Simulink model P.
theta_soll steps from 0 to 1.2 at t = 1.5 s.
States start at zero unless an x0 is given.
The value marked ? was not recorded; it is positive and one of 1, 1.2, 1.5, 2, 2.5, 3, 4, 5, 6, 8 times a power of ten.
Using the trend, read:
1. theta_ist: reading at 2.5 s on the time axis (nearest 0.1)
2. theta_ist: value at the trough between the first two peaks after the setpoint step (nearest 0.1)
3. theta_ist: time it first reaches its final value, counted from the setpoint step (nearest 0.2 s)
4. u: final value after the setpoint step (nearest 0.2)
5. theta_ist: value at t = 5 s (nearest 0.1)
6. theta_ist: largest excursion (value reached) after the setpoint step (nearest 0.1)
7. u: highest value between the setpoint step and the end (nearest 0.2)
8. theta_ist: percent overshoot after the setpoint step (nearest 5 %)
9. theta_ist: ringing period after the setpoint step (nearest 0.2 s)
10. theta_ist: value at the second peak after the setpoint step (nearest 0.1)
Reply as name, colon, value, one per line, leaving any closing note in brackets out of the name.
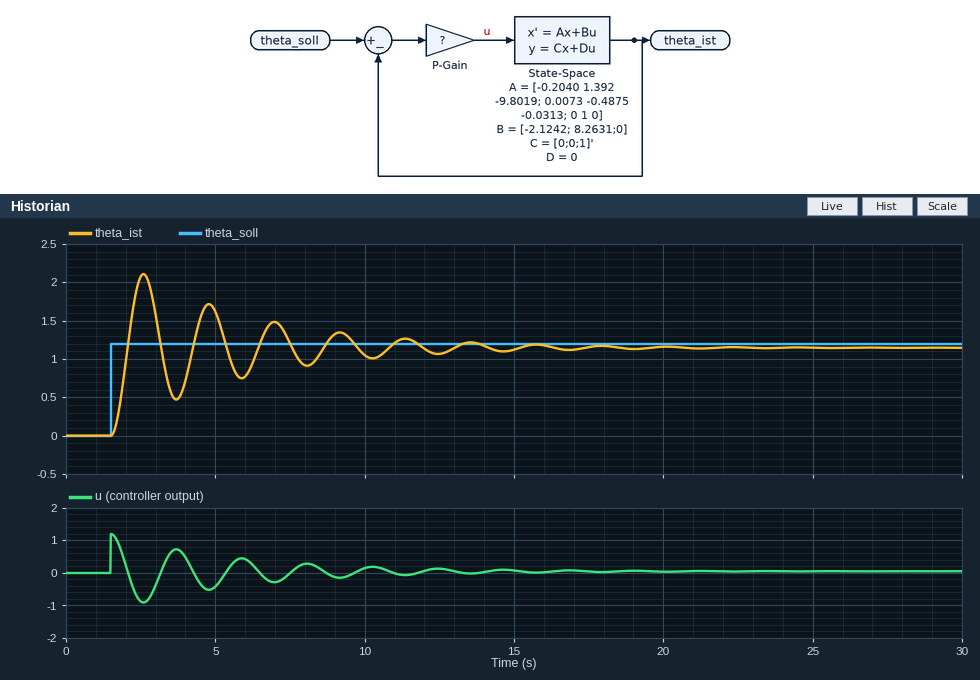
theta_ist: reading at 2.5 s on the time axis: 2.1
theta_ist: value at the trough between the first two peaks after the setpoint step: 0.5
theta_ist: time it first reaches its final value, counted from the setpoint step: 0.6 s
u: final value after the setpoint step: 0.0
theta_ist: value at t = 5 s: 1.6
theta_ist: largest excursion (value reached) after the setpoint step: 2.1
u: highest value between the setpoint step and the end: 1.2
theta_ist: percent overshoot after the setpoint step: 85 %
theta_ist: ringing period after the setpoint step: 2.2 s
theta_ist: value at the second peak after the setpoint step: 1.7
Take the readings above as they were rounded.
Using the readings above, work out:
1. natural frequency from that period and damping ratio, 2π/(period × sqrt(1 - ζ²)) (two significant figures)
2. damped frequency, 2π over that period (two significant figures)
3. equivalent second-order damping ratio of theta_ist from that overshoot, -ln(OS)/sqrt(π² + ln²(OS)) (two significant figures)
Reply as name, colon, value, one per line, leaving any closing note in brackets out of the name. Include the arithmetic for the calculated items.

natural frequency from that period and damping ratio, 2π/(period × sqrt(1 - ζ²)): 2π / (2.2 × sqrt(1 - 0.052²)) = 2.9 rad/s
damped frequency, 2π over that period: 2π / 2.2 = 2.9 rad/s
equivalent second-order damping ratio of theta_ist from that overshoot, -ln(OS)/sqrt(π² + ln²(OS)): ln(0.85) = -0.163; 0.163 / sqrt(9.870 + 0.026) = 0.052
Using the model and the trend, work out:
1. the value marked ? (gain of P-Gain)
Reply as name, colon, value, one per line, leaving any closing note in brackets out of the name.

the value marked ?: 1
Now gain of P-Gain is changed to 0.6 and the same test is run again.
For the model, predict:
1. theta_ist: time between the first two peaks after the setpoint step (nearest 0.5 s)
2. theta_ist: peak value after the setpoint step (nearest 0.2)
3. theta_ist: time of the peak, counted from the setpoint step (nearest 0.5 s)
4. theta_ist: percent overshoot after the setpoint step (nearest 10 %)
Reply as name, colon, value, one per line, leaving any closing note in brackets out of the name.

theta_ist: time between the first two peaks after the setpoint step: 3.0 s
theta_ist: peak value after the setpoint step: 2.0
theta_ist: time of the peak, counted from the setpoint step: 1.5 s
theta_ist: percent overshoot after the setpoint step: 80 %
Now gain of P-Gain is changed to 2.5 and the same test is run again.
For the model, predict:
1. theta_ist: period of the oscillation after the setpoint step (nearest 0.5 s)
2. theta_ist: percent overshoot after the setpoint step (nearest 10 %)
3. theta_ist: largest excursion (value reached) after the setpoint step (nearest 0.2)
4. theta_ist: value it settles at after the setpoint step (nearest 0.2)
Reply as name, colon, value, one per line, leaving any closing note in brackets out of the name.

theta_ist: period of the oscillation after the setpoint step: 1.5 s
theta_ist: percent overshoot after the setpoint step: 90 %
theta_ist: largest excursion (value reached) after the setpoint step: 2.2
theta_ist: value it settles at after the setpoint step: 1.2
